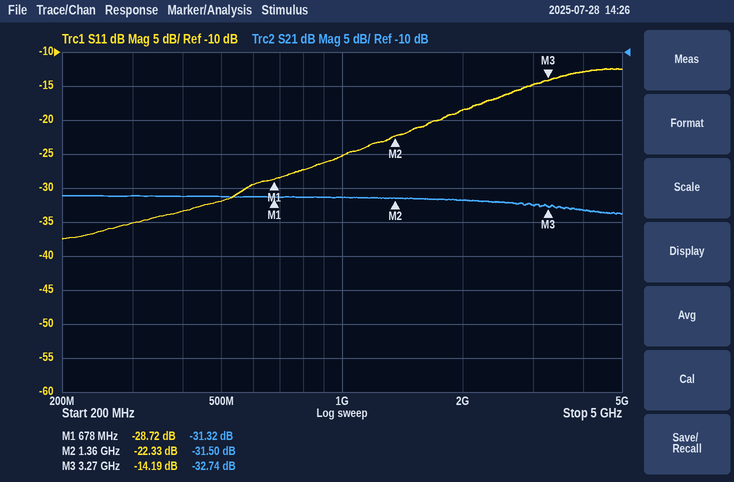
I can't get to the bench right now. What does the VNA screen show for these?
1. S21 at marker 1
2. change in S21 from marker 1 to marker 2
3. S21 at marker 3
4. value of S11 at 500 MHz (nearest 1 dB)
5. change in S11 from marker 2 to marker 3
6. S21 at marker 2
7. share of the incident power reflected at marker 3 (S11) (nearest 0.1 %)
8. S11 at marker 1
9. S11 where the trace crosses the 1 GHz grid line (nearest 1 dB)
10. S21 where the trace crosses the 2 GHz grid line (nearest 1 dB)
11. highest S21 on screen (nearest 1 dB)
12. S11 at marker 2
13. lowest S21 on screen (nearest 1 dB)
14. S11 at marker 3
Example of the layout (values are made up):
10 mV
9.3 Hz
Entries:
-31.32 dB
-0.18 dB
-32.74 dB
-32 dB
8.14 dB
-31.50 dB
3.8 %
-28.72 dB
-25 dB
-32 dB
-31 dB
-22.33 dB
-34 dB
-14.19 dB
